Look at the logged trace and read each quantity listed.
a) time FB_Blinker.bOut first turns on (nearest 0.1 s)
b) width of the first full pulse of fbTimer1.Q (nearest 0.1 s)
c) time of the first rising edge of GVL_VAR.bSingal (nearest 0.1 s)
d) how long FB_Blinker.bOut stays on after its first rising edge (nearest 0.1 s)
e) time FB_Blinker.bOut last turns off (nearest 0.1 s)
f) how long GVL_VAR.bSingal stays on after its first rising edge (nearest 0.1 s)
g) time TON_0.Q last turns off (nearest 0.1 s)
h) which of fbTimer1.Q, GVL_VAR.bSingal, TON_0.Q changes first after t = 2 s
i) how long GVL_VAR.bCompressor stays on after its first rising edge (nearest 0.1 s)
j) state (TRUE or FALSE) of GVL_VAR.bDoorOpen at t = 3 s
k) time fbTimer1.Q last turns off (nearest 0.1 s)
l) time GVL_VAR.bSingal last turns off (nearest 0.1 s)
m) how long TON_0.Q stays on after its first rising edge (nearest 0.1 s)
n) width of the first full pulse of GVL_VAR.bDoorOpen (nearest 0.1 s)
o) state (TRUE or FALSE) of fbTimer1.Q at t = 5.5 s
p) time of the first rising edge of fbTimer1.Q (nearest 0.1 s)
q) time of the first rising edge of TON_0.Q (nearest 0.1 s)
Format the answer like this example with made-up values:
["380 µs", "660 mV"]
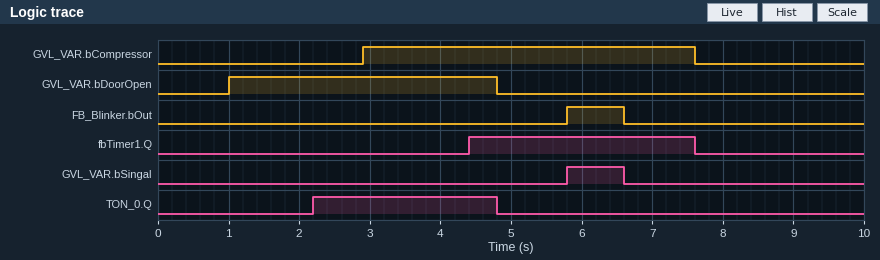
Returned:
["5.8 s", "3.2 s", "5.8 s", "0.8 s", "6.6 s", "0.8 s", "4.8 s", "TON_0.Q", "4.7 s", "TRUE", "7.6 s", "6.6 s", "2.6 s", "3.8 s", "TRUE", "4.4 s", "2.2 s"]
